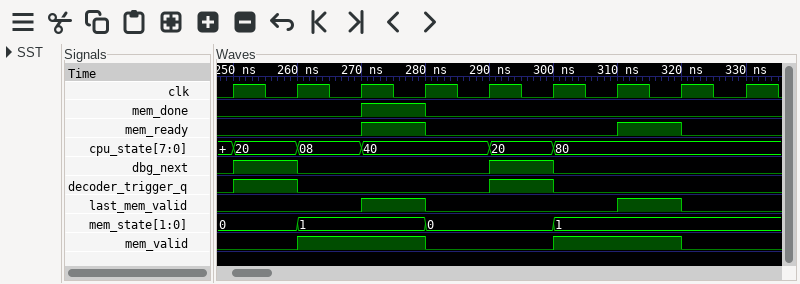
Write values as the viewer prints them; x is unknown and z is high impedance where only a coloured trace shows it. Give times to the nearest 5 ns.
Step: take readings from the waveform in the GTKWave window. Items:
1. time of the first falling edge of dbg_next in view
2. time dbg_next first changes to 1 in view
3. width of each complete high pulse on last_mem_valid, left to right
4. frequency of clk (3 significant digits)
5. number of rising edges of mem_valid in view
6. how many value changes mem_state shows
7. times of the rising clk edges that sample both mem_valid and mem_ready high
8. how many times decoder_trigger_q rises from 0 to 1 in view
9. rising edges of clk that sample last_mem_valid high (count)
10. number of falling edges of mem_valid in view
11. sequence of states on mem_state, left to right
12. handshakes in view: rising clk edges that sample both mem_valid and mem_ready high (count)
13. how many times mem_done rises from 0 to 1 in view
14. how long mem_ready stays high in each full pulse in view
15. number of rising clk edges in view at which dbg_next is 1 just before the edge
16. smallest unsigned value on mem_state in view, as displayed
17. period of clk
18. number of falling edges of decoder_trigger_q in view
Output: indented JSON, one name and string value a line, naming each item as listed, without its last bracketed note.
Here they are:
{
  "time of the first falling edge of dbg_next in view": "260 ns",
  "time dbg_next first changes to 1 in view": "250 ns",
  "width of each complete high pulse on last_mem_valid, left to right": "10 ns, 10 ns",
  "frequency of clk": "100 MHz",
  "number of rising edges of mem_valid in view": "2",
  "how many value changes mem_state shows": "3",
  "times of the rising clk edges that sample both mem_valid and mem_ready high": "280 ns, 320 ns",
  "how many times decoder_trigger_q rises from 0 to 1 in view": "2",
  "rising edges of clk that sample last_mem_valid high": "2",
  "number of falling edges of mem_valid in view": "2",
  "sequence of states on mem_state, left to right": "0, 1, 0, 1",
  "handshakes in view: rising clk edges that sample both mem_valid and mem_ready high": "2",
  "how many times mem_done rises from 0 to 1 in view": "1",
  "how long mem_ready stays high in each full pulse in view": "10 ns, 10 ns",
  "number of rising clk edges in view at which dbg_next is 1 just before the edge": "2",
  "smallest unsigned value on mem_state in view, as displayed": "0",
  "period of clk": "10 ns",
  "number of falling edges of decoder_trigger_q in view": "2"
}
